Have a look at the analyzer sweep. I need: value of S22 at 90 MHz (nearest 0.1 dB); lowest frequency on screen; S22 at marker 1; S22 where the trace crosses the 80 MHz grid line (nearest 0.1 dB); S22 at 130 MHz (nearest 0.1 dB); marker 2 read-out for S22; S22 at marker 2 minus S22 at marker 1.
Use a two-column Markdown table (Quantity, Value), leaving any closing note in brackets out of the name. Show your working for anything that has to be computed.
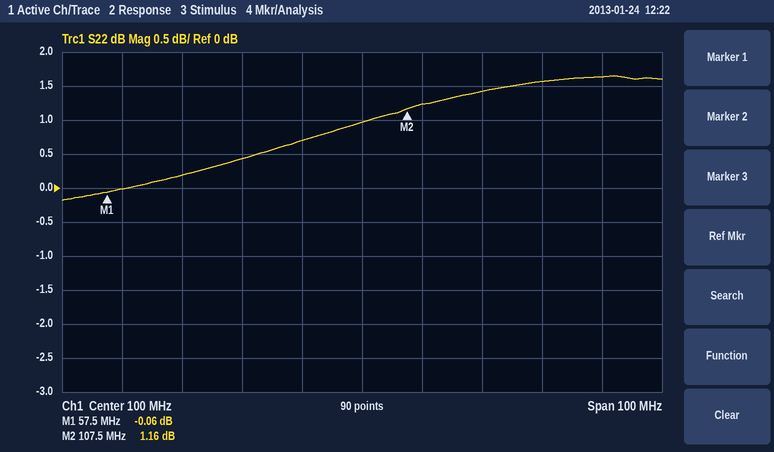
| Quantity | Value |
|---|---|
| value of S22 at 90 MHz | 0.7 dB |
| lowest frequency on screen | 50 MHz |
| S22 at marker 1 | -0.06 dB |
| S22 where the trace crosses the 80 MHz grid line | 0.4 dB |
| S22 at 130 MHz | 1.6 dB |
| marker 2 read-out for S22 | 1.16 dB |
| S22 at marker 2 minus S22 at marker 1 | 1.16 − (-0.06) = 1.22 dB |
